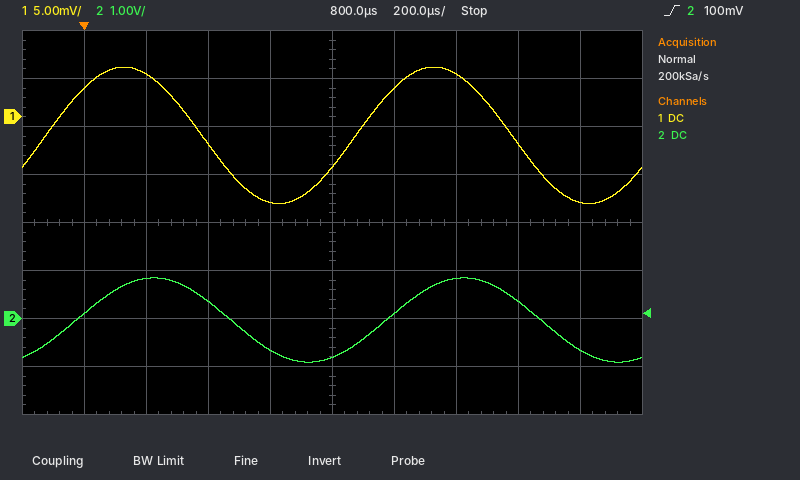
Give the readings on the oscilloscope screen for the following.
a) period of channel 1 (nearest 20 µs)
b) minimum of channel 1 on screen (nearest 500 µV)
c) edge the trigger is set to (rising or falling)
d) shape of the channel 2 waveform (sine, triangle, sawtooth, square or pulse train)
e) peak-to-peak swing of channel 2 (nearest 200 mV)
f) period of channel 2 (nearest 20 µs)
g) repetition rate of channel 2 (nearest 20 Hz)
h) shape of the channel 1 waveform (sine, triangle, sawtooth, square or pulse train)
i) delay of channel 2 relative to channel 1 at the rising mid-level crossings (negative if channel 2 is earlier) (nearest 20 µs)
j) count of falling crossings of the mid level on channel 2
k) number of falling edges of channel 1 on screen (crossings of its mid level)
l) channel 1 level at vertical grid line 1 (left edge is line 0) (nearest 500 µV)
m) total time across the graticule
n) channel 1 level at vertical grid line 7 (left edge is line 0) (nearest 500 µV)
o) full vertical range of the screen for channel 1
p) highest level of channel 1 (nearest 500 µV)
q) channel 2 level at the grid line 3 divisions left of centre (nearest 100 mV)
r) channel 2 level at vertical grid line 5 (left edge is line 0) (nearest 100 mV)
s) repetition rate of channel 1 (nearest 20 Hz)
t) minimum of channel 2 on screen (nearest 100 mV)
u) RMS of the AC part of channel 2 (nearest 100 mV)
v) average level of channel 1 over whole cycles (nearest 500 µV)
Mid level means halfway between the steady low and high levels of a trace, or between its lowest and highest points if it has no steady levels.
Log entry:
1.00 ms
-9.0 mV
rising
sine
1.8 V
1.00 ms
1.00 kHz
sine
+100 µs
2
2
3.0 mV
2 ms
4.5 mV
40 mV
5.0 mV
800 mV
-800 mV
1.00 kHz
-900 mV
600 mV
-2.0 mV
